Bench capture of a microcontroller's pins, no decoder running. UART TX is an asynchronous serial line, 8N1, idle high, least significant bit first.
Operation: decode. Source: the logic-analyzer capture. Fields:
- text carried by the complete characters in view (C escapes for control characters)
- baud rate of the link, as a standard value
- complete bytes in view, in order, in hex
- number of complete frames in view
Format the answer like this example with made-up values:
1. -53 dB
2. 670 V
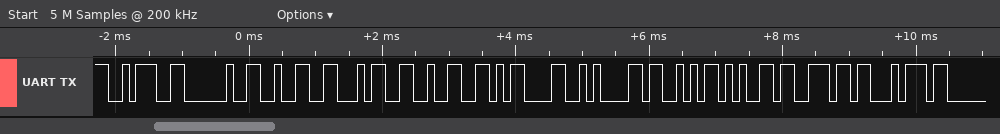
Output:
1. ": 242\r\nSent"
2. 9600 baud
3. 3A 20 32 34 32 0D 0A 53 65 6E 74
4. 11
